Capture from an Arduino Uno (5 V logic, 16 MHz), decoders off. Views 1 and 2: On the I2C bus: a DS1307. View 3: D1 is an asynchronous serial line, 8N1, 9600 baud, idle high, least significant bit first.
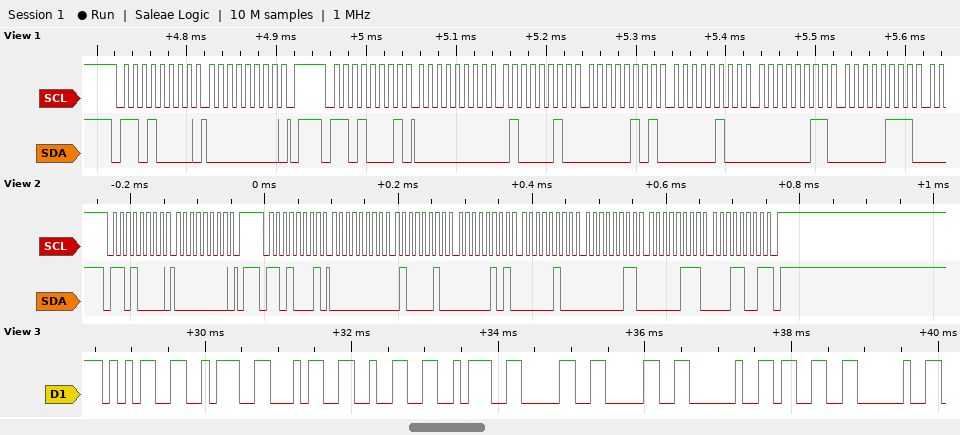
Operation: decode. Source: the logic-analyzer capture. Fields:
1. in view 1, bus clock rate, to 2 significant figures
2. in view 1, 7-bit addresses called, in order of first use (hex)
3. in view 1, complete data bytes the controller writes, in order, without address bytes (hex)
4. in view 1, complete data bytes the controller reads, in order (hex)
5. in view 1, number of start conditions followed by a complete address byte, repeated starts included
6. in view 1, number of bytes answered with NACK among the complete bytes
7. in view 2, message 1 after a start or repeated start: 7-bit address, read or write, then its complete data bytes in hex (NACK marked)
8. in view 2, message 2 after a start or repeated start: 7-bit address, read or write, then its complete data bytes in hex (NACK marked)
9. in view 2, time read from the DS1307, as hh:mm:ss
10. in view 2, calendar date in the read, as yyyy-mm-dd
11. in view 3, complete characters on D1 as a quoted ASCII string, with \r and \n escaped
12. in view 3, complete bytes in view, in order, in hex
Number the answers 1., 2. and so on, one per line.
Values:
1. 100 kHz
2. 0x68
3. 00
4. 00 42 05 04 03 07
5. 2
6. 0
7. 0x68 write: 00
8. 0x68 read: 00 42 05 04 03 07 19 NACK
9. 05:42:00
10. 2019-07-03
11. "5:42:00 3 "
12. 35 3A 34 32 3A 30 30 20 33 20
